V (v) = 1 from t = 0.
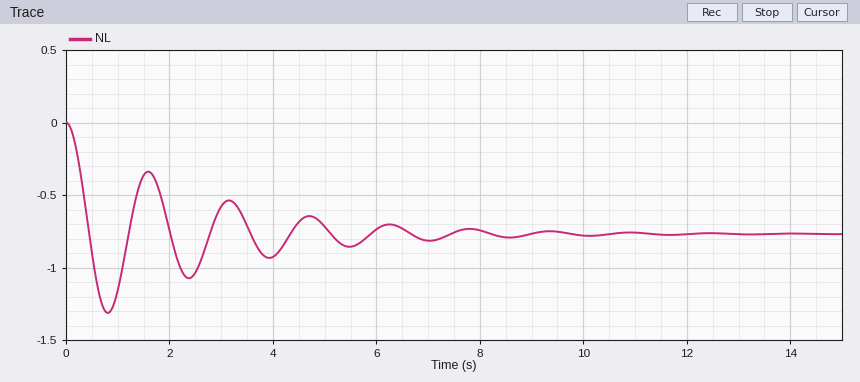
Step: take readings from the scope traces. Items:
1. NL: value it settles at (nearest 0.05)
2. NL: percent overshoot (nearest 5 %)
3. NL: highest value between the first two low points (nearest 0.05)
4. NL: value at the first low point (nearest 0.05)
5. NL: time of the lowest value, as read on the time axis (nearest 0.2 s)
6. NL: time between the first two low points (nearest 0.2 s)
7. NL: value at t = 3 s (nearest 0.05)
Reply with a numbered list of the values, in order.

1. -0.75
2. 70 %
3. -0.35
4. -1.30
5. 0.8 s
6. 1.6 s
7. -0.60
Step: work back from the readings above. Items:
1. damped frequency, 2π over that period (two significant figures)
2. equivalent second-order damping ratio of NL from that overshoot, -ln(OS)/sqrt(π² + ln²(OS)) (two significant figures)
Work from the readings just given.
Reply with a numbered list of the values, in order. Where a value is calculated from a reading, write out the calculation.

1. 2π / 1.6 = 3.9 rad/s
2. ln(0.7) = -0.357; 0.357 / sqrt(9.870 + 0.127) = 0.11
